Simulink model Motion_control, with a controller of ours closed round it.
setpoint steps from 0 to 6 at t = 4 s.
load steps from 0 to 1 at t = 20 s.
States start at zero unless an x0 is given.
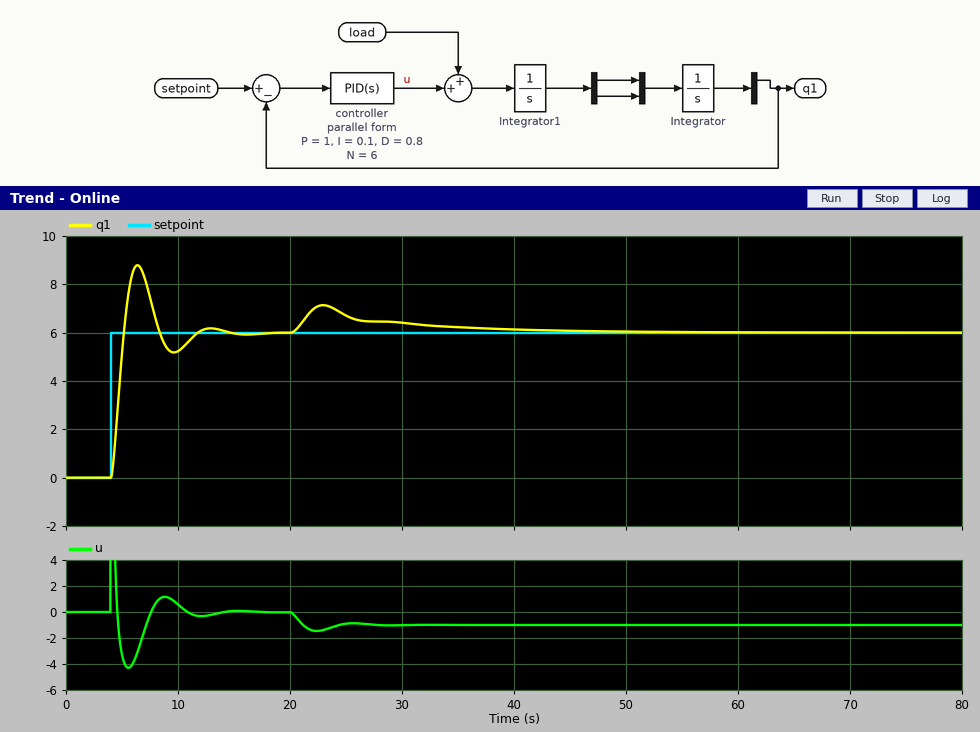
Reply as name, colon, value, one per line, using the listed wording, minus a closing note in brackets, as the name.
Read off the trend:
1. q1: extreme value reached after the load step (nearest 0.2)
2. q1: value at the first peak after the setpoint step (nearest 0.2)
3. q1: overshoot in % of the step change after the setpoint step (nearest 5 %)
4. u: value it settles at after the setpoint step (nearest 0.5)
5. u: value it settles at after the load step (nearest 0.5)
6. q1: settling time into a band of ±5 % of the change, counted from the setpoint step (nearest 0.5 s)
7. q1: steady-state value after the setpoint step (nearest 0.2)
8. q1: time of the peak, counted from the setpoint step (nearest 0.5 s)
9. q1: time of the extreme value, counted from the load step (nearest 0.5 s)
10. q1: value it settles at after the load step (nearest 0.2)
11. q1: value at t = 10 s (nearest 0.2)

q1: extreme value reached after the load step: 7.2
q1: value at the first peak after the setpoint step: 8.8
q1: overshoot in % of the step change after the setpoint step: 45 %
u: value it settles at after the setpoint step: 0.0
u: value it settles at after the load step: -1.0
q1: settling time into a band of ±5 % of the change, counted from the setpoint step: 7.0 s
q1: steady-state value after the setpoint step: 6.0
q1: time of the peak, counted from the setpoint step: 2.5 s
q1: time of the extreme value, counted from the load step: 3.0 s
q1: value it settles at after the load step: 6.0
q1: value at t = 10 s: 5.2
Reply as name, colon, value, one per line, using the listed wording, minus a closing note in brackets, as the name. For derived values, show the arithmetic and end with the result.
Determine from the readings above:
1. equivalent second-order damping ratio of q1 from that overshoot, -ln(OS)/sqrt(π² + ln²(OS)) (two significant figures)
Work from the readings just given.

equivalent second-order damping ratio of q1 from that overshoot, -ln(OS)/sqrt(π² + ln²(OS)): ln(0.45) = -0.799; 0.799 / sqrt(9.870 + 0.638) = 0.25
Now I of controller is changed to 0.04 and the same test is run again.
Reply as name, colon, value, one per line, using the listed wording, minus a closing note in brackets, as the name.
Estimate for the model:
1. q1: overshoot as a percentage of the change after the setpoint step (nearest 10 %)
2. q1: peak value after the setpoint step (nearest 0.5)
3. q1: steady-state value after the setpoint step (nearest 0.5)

q1: overshoot as a percentage of the change after the setpoint step: 40 %
q1: peak value after the setpoint step: 8.5
q1: steady-state value after the setpoint step: 6.0
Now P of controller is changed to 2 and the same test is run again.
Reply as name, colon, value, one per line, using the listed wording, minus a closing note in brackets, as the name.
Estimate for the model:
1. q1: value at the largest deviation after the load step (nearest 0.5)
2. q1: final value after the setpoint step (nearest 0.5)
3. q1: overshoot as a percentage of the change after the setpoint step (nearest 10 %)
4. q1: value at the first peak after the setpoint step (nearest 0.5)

q1: value at the largest deviation after the load step: 6.5
q1: final value after the setpoint step: 6.0
q1: overshoot as a percentage of the change after the setpoint step: 60 %
q1: value at the first peak after the setpoint step: 9.5
